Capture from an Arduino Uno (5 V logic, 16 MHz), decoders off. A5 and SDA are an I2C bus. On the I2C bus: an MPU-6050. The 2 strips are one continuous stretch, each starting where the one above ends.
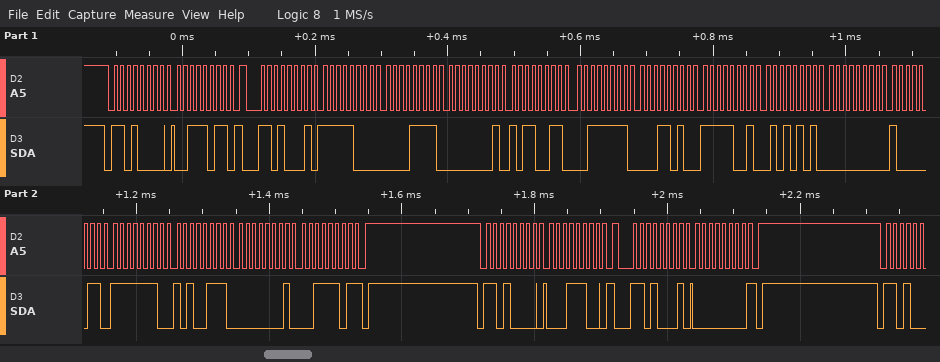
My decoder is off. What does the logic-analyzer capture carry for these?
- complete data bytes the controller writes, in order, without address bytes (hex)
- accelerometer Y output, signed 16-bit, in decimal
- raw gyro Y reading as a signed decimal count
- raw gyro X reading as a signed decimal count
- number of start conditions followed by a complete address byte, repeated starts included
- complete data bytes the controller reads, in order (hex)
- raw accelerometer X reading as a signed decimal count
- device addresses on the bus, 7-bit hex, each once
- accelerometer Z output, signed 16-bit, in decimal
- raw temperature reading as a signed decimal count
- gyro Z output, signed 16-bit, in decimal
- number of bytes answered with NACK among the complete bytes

3B 1C
435
-345
131
4
F8 0F 01 B3 3F 1A F9 55 00 83 FE A7 01 3D 00
-2033
0x68
16154
-1707
317
2
